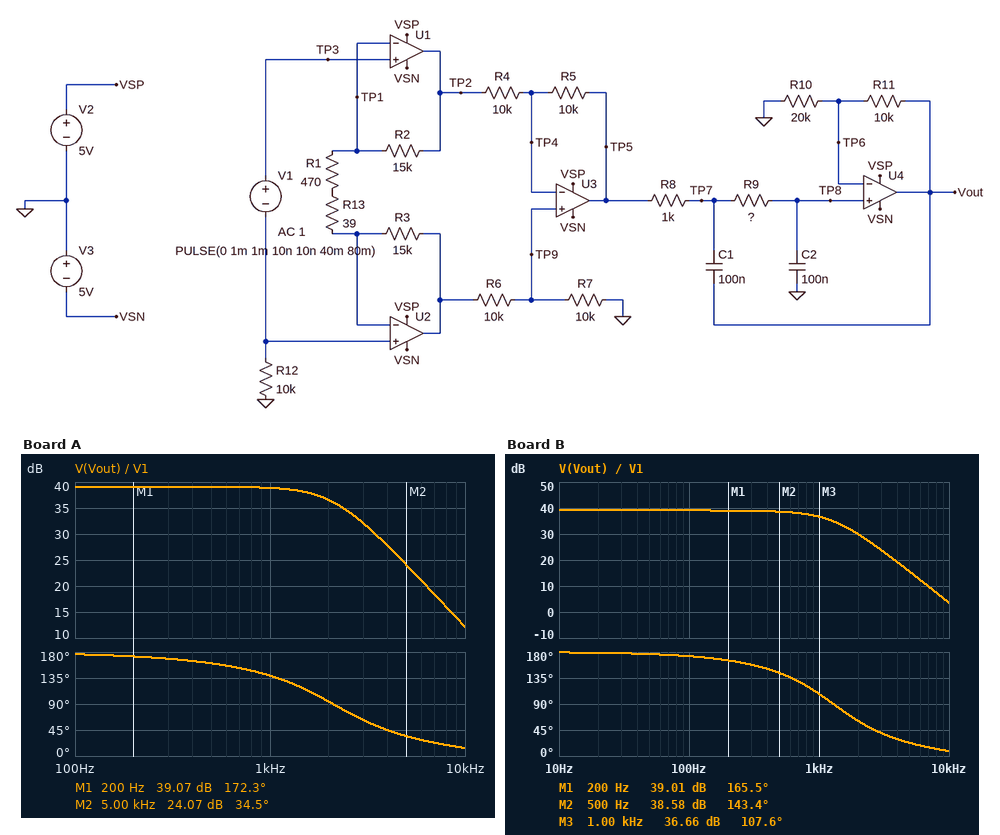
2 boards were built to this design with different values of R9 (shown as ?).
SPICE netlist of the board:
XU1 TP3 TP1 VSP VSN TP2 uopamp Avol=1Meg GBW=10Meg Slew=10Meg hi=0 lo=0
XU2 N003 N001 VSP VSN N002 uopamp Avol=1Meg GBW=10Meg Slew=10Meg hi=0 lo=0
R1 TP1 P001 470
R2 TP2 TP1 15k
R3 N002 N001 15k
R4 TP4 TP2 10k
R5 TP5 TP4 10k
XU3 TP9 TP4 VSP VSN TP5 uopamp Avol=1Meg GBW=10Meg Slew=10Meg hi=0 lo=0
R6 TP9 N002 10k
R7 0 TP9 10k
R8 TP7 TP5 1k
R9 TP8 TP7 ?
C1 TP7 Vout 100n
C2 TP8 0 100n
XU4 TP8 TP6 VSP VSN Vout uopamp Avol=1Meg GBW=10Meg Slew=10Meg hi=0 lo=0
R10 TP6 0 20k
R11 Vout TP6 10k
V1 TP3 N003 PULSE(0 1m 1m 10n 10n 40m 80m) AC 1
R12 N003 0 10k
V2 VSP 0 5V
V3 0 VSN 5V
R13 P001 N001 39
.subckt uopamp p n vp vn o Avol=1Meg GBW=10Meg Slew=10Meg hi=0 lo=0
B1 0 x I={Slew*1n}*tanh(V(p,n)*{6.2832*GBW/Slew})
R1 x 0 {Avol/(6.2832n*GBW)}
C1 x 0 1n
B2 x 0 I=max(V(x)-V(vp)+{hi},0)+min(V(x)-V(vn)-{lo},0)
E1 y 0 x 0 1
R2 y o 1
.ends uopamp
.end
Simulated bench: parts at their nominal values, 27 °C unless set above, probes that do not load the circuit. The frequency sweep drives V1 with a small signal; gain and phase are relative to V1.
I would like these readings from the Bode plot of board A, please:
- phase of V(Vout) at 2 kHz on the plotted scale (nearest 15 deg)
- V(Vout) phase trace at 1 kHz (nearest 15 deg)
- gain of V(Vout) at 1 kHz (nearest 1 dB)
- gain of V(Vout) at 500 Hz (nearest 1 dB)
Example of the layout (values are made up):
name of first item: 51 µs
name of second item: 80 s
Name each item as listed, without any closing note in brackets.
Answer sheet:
phase of V(Vout) at 2 kHz on the plotted scale: 90 deg
V(Vout) phase trace at 1 kHz: 135 deg
gain of V(Vout) at 1 kHz: 39 dB
gain of V(Vout) at 500 Hz: 39 dB
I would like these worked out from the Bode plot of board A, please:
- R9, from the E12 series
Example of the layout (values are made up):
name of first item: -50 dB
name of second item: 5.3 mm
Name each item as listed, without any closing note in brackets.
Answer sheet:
R9, from the E12 series: 560 Ω
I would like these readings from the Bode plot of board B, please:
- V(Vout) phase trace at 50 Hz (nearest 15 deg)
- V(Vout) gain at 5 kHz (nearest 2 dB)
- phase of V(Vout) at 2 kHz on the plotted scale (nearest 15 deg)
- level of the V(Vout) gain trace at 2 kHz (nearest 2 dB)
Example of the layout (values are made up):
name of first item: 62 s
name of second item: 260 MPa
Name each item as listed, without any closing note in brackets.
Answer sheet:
V(Vout) phase trace at 50 Hz: 180 deg
V(Vout) gain at 5 kHz: 16 dB
phase of V(Vout) at 2 kHz on the plotted scale: 60 deg
level of the V(Vout) gain trace at 2 kHz: 30 dB
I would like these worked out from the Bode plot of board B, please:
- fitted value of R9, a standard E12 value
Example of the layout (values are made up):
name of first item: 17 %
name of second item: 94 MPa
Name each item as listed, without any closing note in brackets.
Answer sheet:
fitted value of R9, a standard E12 value: 1.5 kΩ
